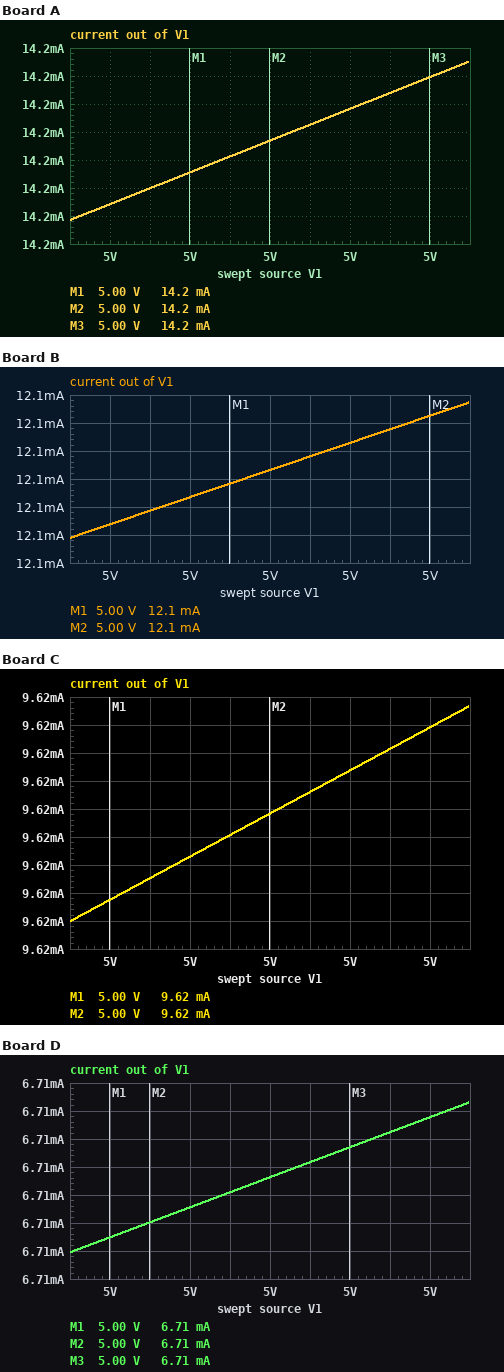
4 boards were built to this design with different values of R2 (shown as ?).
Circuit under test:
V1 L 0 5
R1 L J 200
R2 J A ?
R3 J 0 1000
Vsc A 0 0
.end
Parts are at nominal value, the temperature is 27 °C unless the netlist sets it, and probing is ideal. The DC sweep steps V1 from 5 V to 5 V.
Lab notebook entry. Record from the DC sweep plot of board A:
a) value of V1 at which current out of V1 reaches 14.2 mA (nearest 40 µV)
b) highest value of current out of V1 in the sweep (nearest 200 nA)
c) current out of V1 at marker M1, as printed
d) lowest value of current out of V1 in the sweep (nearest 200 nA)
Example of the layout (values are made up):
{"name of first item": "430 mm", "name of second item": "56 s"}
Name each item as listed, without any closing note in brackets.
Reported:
{"value of V1 at which current out of V1 reaches 14.2 mA": "4.99940 V", "highest value of current out of V1 in the sweep": "14.1856 mA", "current out of V1 at marker M1, as printed": "14.2 mA", "lowest value of current out of V1 in the sweep": "14.1798 mA"}
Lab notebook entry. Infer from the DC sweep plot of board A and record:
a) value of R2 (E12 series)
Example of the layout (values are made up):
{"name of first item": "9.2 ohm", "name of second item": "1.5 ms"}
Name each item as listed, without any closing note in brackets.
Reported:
{"value of R2": "180 Ω"}
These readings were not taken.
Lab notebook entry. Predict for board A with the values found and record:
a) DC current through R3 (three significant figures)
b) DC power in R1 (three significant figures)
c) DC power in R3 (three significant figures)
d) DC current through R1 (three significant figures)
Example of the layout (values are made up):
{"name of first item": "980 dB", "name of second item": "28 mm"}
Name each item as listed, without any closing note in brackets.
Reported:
{"DC current through R3": "2.16 mA", "DC power in R1": "40.2 mW", "DC power in R3": "4.68 mW", "DC current through R1": "14.2 mA"}
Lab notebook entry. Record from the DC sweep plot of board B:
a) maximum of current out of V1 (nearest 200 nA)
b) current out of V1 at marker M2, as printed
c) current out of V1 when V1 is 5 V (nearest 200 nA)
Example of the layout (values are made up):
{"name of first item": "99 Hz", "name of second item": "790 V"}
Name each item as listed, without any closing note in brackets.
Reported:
{"maximum of current out of V1": "12.1208 mA", "current out of V1 at marker M2, as printed": "12.1 mA", "current out of V1 when V1 is 5 V": "12.1178 mA"}
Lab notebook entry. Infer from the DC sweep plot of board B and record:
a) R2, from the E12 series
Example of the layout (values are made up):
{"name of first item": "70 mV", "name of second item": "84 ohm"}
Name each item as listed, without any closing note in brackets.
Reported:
{"R2, from the E12 series": "270 Ω"}
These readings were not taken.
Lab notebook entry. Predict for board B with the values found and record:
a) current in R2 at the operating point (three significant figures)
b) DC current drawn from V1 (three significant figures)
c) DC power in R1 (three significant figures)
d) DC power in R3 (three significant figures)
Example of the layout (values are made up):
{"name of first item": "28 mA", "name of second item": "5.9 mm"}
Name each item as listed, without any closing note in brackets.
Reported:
{"current in R2 at the operating point": "9.54 mA", "DC current drawn from V1": "12.1 mA", "DC power in R1": "29.4 mW", "DC power in R3": "6.64 mW"}
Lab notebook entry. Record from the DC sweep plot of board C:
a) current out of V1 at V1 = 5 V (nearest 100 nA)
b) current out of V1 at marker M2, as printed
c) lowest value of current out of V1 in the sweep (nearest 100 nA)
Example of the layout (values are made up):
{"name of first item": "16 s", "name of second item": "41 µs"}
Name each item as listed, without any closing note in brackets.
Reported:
{"current out of V1 at V1 = 5 V": "9.6200 mA", "current out of V1 at marker M2, as printed": "9.62 mA", "lowest value of current out of V1 in the sweep": "9.6185 mA"}
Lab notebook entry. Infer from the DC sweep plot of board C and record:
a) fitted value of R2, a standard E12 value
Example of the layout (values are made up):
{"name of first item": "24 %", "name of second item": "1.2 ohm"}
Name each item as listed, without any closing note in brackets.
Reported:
{"fitted value of R2, a standard E12 value": "470 Ω"}
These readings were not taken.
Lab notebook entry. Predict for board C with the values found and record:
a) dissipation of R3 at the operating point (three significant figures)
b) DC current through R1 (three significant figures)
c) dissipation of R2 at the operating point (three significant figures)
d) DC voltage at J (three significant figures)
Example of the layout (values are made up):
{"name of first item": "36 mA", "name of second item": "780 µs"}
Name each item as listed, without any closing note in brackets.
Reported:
{"dissipation of R3 at the operating point": "9.46 mW", "DC current through R1": "9.62 mA", "dissipation of R2 at the operating point": "20.1 mW", "DC voltage at J": "3.08 V"}
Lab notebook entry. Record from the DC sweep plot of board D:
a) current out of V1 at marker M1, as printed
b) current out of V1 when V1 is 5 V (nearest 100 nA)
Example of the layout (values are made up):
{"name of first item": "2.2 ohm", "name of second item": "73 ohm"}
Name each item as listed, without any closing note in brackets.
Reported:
{"current out of V1 at marker M1, as printed": "6.71 mA", "current out of V1 when V1 is 5 V": "6.7065 mA"}
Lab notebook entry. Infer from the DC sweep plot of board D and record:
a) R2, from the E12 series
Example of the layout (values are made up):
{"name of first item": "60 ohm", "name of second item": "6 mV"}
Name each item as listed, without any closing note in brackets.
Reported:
{"R2, from the E12 series": "1.2 kΩ"}
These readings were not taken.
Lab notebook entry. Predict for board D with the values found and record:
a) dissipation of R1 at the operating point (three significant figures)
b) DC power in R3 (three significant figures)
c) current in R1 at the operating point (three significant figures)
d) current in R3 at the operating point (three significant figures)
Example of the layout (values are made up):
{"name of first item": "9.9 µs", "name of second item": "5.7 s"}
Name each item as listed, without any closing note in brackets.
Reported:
{"dissipation of R1 at the operating point": "9.00 mW", "DC power in R3": "13.4 mW", "current in R1 at the operating point": "6.71 mA", "current in R3 at the operating point": "3.66 mA"}
